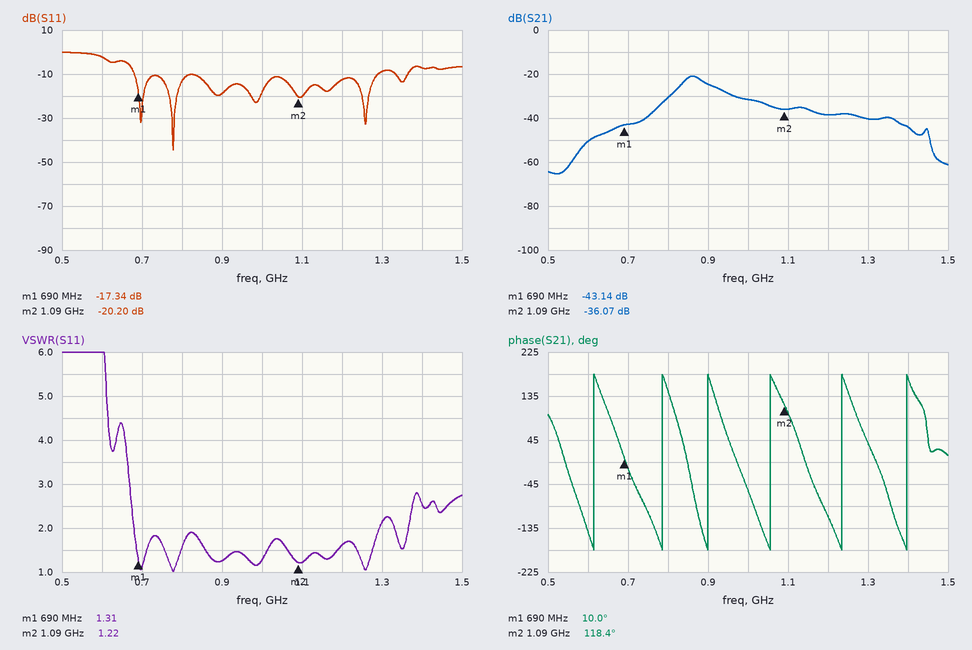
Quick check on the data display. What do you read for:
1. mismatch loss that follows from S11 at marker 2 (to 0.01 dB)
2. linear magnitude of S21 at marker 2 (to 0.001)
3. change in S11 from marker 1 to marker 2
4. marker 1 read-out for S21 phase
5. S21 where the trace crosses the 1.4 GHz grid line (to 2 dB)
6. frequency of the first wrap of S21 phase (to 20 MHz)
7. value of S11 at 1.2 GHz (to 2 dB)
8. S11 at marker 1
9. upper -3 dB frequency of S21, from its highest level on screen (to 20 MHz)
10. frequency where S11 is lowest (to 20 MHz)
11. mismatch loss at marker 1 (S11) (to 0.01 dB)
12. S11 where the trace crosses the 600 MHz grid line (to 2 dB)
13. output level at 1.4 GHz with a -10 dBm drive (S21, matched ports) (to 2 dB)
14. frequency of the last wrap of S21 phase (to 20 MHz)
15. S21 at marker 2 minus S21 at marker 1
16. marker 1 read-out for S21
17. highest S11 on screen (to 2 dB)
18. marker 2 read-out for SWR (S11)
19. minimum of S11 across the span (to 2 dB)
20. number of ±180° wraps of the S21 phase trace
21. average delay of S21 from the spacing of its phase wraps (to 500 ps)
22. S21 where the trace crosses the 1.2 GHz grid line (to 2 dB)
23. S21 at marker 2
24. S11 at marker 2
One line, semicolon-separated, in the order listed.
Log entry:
0.04 dB; 0.016; -2.86 dB; 10.0°; -44 dB; 620 MHz; -12 dB; -17.34 dB; 900 MHz; 780 MHz; 0.08 dB; -2 dB; -54 dBm; 1.40 GHz; 7.07 dB; -43.14 dB; 0 dB; 1.22; -44 dB; 6; 6.5 ns; -38 dB; -36.07 dB; -20.20 dB
